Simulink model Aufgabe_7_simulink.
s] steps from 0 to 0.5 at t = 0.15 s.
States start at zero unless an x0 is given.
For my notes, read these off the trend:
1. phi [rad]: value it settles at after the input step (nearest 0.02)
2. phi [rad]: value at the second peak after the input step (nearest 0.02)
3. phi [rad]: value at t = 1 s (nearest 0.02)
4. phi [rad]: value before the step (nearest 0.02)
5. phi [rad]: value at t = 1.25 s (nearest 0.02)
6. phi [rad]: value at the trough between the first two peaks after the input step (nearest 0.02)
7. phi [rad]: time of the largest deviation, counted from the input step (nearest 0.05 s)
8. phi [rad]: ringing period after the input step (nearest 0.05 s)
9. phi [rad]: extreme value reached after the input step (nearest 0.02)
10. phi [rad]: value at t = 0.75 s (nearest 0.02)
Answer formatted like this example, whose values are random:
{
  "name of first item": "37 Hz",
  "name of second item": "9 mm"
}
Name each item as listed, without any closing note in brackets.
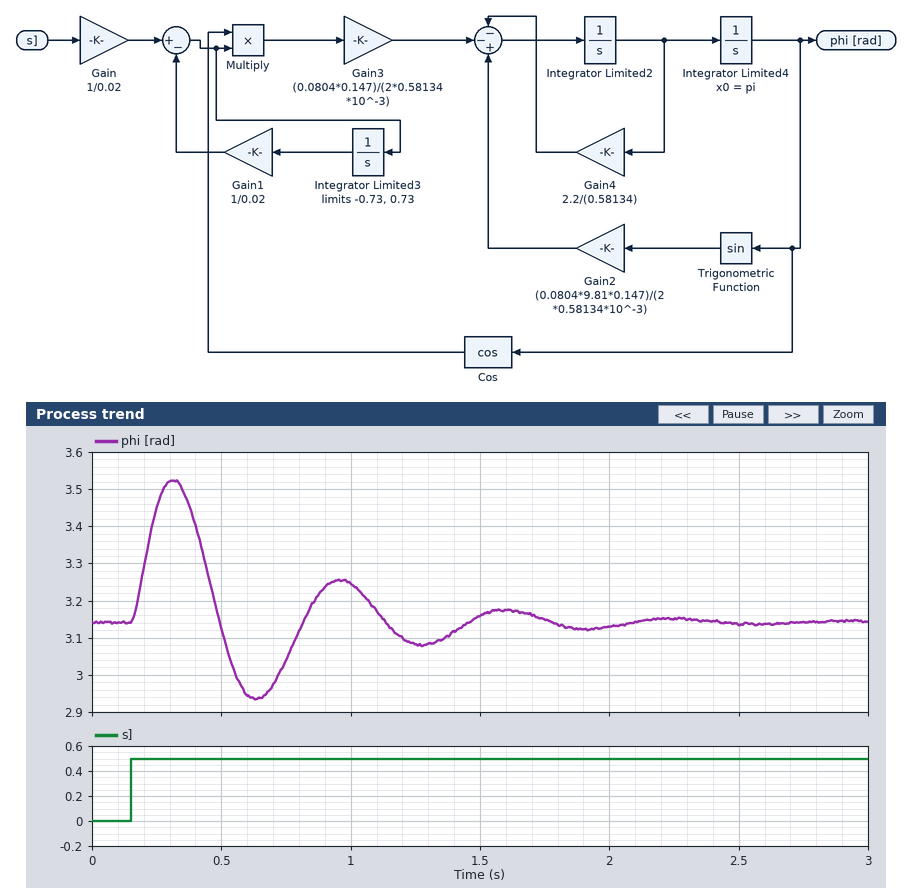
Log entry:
{
  "phi [rad]: value it settles at after the input step": "3.14",
  "phi [rad]: value at the second peak after the input step": "3.26",
  "phi [rad]: value at t = 1 s": "3.24",
  "phi [rad]: value before the step": "3.14",
  "phi [rad]: value at t = 1.25 s": "3.08",
  "phi [rad]: value at the trough between the first two peaks after the input step": "2.94",
  "phi [rad]: time of the largest deviation, counted from the input step": "0.15 s",
  "phi [rad]: ringing period after the input step": "0.65 s",
  "phi [rad]: extreme value reached after the input step": "3.52",
  "phi [rad]: value at t = 0.75 s": "3.04"
}
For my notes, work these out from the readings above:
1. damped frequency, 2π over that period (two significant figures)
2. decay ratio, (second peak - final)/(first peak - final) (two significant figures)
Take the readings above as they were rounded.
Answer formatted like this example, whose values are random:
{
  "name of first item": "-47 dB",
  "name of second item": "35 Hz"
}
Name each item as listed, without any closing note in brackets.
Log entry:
{
  "damped frequency, 2π over that period": "9.7 rad/s",
  "decay ratio, (second peak - final)/(first peak - final)": "0.32"
}
